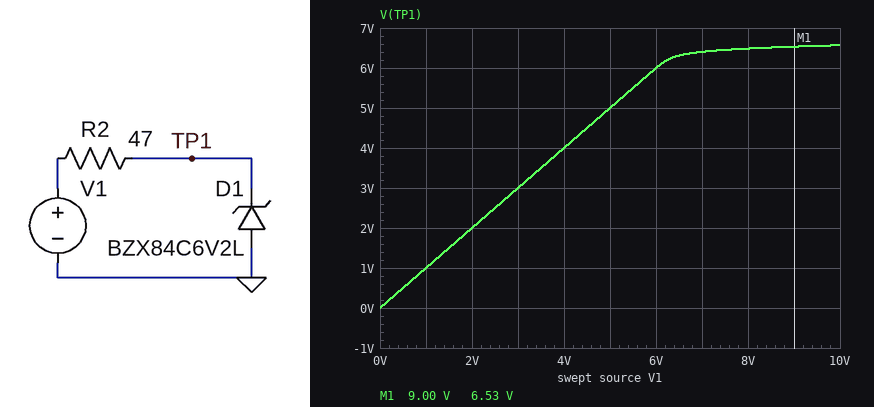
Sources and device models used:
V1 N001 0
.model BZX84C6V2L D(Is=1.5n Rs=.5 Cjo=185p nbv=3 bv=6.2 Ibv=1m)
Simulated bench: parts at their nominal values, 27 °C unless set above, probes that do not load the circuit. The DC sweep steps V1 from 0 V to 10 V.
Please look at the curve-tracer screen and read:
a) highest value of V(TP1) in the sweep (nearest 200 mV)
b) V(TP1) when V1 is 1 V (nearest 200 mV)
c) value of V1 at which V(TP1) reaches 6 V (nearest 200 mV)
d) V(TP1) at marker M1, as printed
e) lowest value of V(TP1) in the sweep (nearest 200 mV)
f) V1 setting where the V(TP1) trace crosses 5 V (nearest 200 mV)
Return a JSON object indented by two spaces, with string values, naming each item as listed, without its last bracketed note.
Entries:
{
  "highest value of V(TP1) in the sweep": "6.6 V",
  "V(TP1) when V1 is 1 V": "1.0 V",
  "value of V1 at which V(TP1) reaches 6 V": "6.0 V",
  "V(TP1) at marker M1, as printed": "6.53 V",
  "lowest value of V(TP1) in the sweep": "0 V",
  "V1 setting where the V(TP1) trace crosses 5 V": "5.0 V"
}
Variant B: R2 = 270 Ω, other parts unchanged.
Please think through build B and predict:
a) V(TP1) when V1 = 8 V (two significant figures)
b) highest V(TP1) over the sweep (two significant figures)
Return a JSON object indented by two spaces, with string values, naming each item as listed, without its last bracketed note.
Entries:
{
  "V(TP1) when V1 = 8 V": "6.3 V",
  "highest V(TP1) over the sweep": "6.4 V"
}
